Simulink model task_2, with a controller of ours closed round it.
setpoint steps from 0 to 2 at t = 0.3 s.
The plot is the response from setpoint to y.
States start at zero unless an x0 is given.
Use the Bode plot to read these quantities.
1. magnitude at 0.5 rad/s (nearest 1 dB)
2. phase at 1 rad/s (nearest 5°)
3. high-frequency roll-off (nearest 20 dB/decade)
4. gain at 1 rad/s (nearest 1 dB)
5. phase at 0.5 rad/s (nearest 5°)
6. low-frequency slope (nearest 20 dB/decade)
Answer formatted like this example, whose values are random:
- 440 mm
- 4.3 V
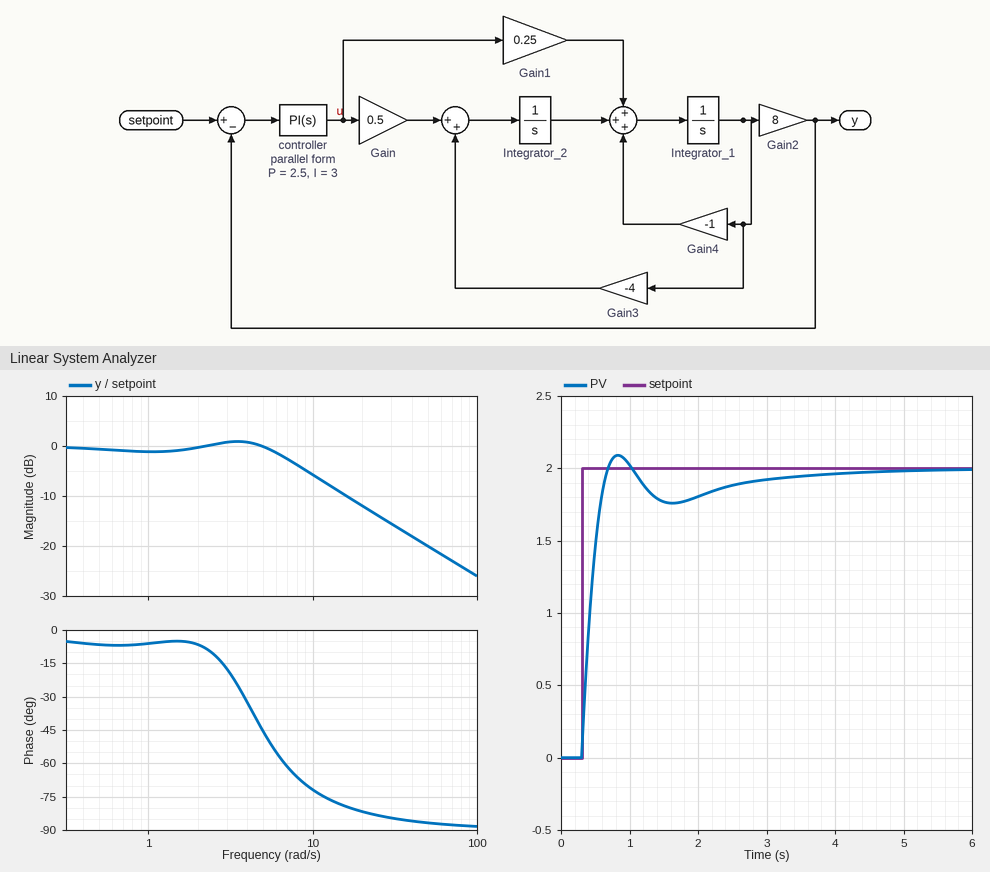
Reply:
- -1 dB
- -5°
- -20 dB/decade
- -1 dB
- -5°
- 0 dB/decade
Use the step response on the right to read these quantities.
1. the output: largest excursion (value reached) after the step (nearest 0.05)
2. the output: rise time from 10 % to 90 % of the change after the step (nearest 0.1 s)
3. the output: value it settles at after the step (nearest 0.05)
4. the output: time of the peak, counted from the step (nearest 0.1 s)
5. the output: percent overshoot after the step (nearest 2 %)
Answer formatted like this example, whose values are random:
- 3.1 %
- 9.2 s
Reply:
- 2.10
- 0.3 s
- 2.00
- 0.5 s
- 4 %
